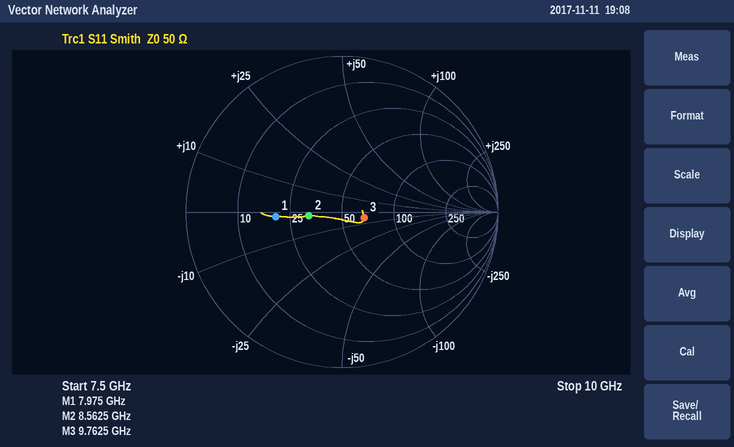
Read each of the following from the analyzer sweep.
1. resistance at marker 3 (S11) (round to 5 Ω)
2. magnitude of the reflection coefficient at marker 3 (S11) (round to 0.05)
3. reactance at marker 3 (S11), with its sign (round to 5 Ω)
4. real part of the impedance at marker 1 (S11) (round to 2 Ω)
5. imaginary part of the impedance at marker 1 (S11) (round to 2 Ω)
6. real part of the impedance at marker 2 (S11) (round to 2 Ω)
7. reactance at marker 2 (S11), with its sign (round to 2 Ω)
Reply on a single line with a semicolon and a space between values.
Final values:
65 Ω; 0.15; -5 Ω; 20 Ω; -2 Ω; 32 Ω; -2 Ω
